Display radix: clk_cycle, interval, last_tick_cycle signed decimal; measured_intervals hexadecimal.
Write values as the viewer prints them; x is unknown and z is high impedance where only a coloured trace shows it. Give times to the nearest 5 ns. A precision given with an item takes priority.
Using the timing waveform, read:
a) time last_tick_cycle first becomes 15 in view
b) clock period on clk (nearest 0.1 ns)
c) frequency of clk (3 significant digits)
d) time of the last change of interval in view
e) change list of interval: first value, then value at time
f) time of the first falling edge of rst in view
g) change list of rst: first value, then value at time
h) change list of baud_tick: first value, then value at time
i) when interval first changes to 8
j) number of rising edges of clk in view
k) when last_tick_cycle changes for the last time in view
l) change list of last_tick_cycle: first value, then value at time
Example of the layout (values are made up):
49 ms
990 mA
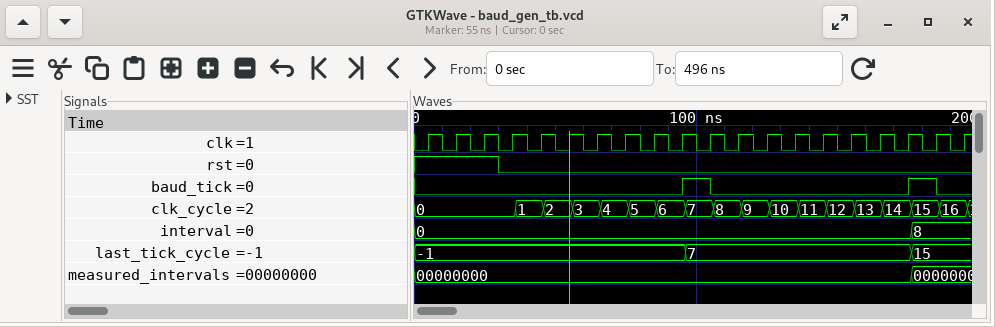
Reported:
175 ns
10 ns
100 MHz
175 ns
0, 8 at 175 ns
30 ns
1, 0 at 30 ns
0, 1 at 95 ns, 0 at 105 ns, 1 at 175 ns, 0 at 185 ns
175 ns
20
175 ns
-1, 7 at 95 ns, 15 at 175 ns
